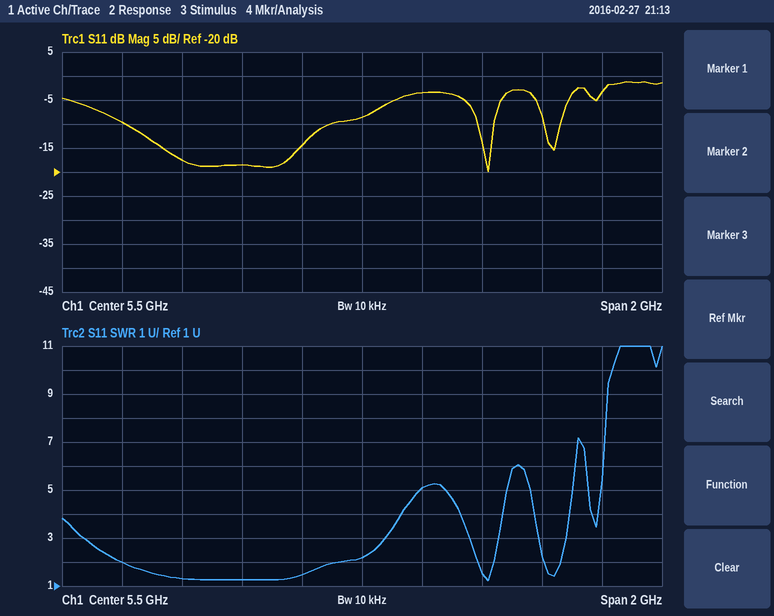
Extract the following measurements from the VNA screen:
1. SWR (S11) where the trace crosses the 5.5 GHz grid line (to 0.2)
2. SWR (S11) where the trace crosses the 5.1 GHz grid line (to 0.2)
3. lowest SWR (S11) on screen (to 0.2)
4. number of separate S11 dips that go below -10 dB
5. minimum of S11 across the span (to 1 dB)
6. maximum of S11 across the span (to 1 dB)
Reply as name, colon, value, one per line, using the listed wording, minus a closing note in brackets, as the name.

SWR (S11) where the trace crosses the 5.5 GHz grid line: 2.2
SWR (S11) where the trace crosses the 5.1 GHz grid line: 1.2
lowest SWR (S11) on screen: 1.2
number of separate S11 dips that go below -10 dB: 3
minimum of S11 across the span: -20 dB
maximum of S11 across the span: -1 dB
